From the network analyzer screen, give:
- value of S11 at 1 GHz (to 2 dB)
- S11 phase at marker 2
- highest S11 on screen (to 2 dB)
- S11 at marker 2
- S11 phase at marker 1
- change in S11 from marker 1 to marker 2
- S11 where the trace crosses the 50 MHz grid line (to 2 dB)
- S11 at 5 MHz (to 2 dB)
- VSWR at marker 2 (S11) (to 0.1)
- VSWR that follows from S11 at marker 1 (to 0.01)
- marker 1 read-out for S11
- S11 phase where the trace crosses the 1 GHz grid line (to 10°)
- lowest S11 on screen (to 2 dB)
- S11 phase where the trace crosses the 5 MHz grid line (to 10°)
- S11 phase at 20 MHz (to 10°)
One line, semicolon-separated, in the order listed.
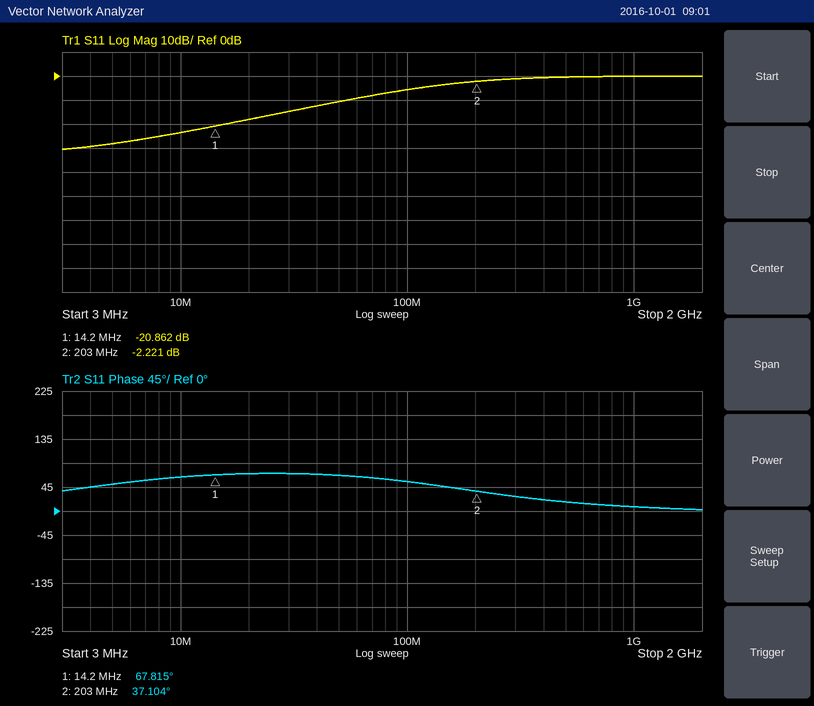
0 dB; 37.104°; 0 dB; -2.221 dB; 67.815°; 18.641 dB; -10 dB; -28 dB; 7.9; 1.20; -20.862 dB; 10°; -30 dB; 50°; 70°
